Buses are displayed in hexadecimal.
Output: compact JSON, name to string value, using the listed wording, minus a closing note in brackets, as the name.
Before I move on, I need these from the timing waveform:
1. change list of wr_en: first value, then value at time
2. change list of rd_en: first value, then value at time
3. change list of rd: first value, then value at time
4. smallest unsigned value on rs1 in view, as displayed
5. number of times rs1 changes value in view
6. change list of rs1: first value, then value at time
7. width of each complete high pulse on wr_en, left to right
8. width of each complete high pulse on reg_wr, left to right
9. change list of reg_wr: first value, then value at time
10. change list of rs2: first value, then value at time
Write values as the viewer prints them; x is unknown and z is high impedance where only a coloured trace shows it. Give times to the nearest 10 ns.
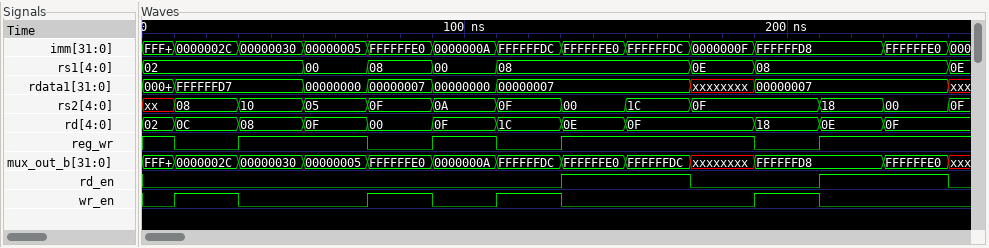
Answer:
{"change list of wr_en: first value, then value at time": "0, 1 at 10 ns, 0 at 30 ns, 1 at 70 ns, 0 at 90 ns, 1 at 110 ns, 0 at 130 ns, 1 at 190 ns, 0 at 210 ns", "change list of rd_en: first value, then value at time": "0, 1 at 130 ns, 0 at 170 ns, 1 at 210 ns, 0 at 250 ns", "change list of rd: first value, then value at time": "02, 0C at 10 ns, 08 at 30 ns, 0F at 50 ns, 00 at 70 ns, 0F at 90 ns, 1C at 110 ns, 0E at 130 ns, 0F at 150 ns, 18 at 190 ns, 0E at 210 ns, 0F at 230 ns", "smallest unsigned value on rs1 in view, as displayed": "00", "number of times rs1 changes value in view": "7", "change list of rs1: first value, then value at time": "02, 00 at 50 ns, 08 at 70 ns, 00 at 90 ns, 08 at 110 ns, 0E at 170 ns, 08 at 190 ns, 0E at 250 ns", "width of each complete high pulse on wr_en, left to right": "20 ns, 20 ns, 20 ns, 20 ns", "width of each complete high pulse on reg_wr, left to right": "40 ns, 20 ns, 60 ns", "change list of reg_wr: first value, then value at time": "1, 0 at 10 ns, 1 at 30 ns, 0 at 70 ns, 1 at 90 ns, 0 at 110 ns, 1 at 130 ns, 0 at 190 ns, 1 at 210 ns", "change list of rs2: first value, then value at time": "xx, 08 at 10 ns, 10 at 30 ns, 05 at 50 ns, 0F at 70 ns, 0A at 90 ns, 0F at 110 ns, 00 at 130 ns, 1C at 150 ns, 0F at 170 ns, 18 at 210 ns, 00 at 230 ns, 0F at 250 ns"}
